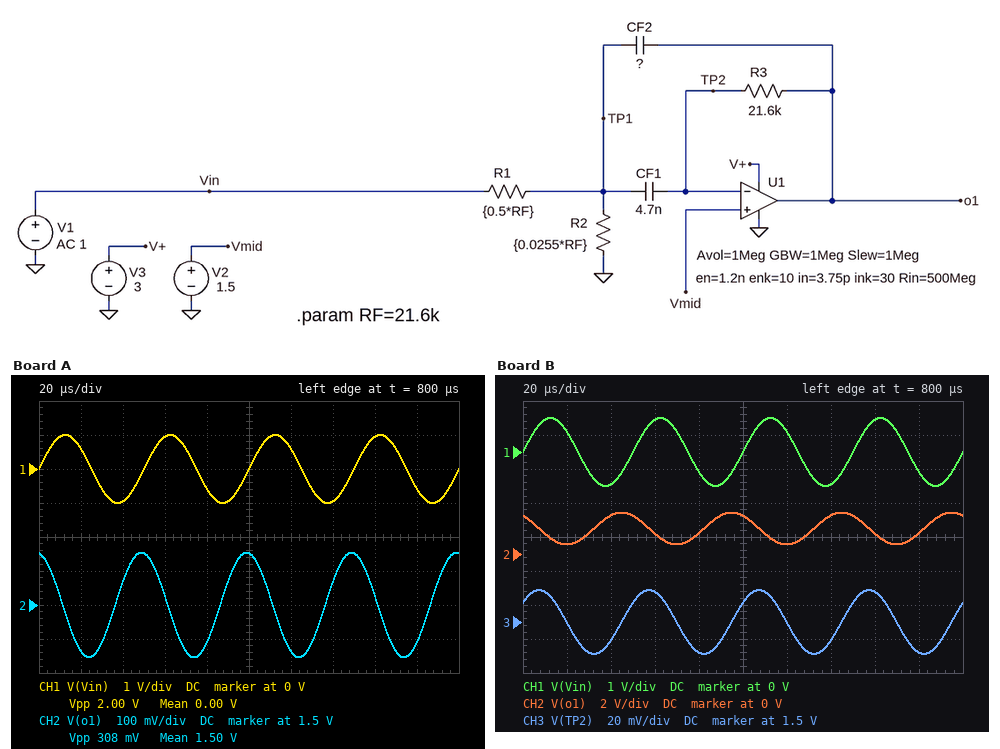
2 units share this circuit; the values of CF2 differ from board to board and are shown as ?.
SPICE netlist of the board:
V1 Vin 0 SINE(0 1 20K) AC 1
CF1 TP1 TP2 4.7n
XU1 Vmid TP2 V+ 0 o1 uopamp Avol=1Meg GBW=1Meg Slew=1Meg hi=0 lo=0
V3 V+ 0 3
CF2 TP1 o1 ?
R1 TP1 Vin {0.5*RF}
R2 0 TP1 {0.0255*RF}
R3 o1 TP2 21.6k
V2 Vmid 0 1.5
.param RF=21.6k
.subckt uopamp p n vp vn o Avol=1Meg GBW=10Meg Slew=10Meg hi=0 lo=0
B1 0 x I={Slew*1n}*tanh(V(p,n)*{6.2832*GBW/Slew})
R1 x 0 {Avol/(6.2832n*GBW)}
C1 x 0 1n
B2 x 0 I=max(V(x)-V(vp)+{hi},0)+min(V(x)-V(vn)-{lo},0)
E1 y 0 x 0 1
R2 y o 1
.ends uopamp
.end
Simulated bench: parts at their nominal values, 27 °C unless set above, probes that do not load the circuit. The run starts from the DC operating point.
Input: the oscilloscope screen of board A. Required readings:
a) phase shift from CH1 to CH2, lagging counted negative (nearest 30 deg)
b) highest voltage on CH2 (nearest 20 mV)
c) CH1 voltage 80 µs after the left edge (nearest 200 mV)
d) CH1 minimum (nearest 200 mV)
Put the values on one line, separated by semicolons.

90 deg; 1.66 V; -600 mV; -1.0 V
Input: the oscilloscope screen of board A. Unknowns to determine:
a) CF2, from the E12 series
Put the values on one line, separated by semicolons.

5.6 nF
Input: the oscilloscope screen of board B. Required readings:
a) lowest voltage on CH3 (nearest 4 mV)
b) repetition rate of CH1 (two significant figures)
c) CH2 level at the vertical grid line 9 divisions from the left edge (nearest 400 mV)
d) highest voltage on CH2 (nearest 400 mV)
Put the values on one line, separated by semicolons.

1.480 V; 20 kHz; 1.2 V; 2.4 V
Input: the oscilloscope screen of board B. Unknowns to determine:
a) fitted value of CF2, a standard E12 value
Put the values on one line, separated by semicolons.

1.5 nF
